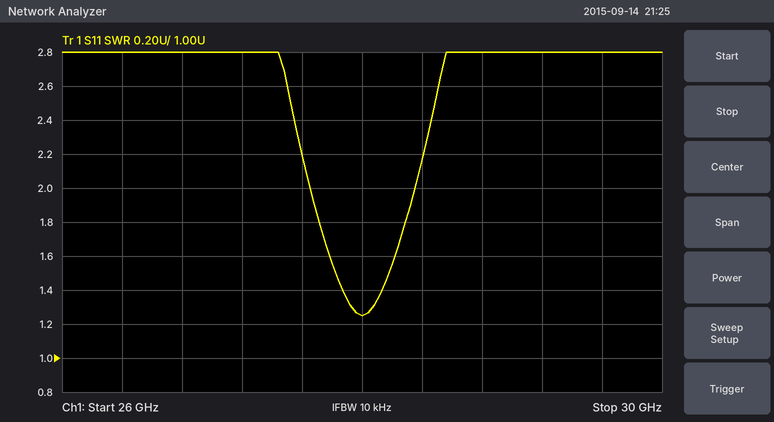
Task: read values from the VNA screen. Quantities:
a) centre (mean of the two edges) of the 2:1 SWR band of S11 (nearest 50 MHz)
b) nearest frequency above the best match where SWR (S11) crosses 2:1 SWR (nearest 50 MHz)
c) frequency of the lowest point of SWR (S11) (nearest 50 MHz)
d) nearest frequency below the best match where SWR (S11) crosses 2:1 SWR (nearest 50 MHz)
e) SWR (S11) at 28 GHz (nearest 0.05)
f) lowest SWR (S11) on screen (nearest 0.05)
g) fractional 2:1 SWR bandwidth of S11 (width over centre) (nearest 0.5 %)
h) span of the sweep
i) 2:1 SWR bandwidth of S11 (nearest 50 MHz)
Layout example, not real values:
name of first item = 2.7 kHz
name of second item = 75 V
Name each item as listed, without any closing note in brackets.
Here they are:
centre (mean of the two edges) of the 2:1 SWR band of S11 = 28.00 GHz
nearest frequency above the best match where SWR (S11) crosses 2:1 SWR = 28.35 GHz
frequency of the lowest point of SWR (S11) = 28.00 GHz
nearest frequency below the best match where SWR (S11) crosses 2:1 SWR = 27.65 GHz
SWR (S11) at 28 GHz = 1.25
lowest SWR (S11) on screen = 1.25
fractional 2:1 SWR bandwidth of S11 (width over centre) = 2.5 %
span of the sweep = 4 GHz
2:1 SWR bandwidth of S11 = 700 MHz
